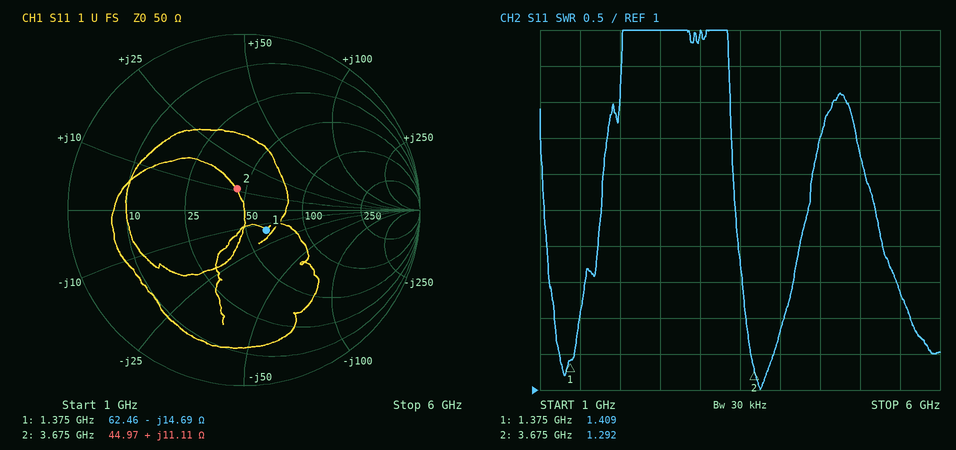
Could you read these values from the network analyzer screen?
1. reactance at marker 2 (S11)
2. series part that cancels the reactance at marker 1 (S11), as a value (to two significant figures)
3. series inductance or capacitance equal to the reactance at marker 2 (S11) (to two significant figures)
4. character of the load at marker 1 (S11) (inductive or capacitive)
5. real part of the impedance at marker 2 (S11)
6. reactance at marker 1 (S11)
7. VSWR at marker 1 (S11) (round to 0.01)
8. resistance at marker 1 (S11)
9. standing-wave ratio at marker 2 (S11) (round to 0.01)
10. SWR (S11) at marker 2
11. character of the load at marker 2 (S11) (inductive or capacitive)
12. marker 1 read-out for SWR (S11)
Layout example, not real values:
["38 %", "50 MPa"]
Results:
["+11.11 Ω", "1.7 nH", "480 pH", "capacitive", "44.97 Ω", "-14.69 Ω", "1.41", "62.46 Ω", "1.29", "1.292", "inductive", "1.409"]
